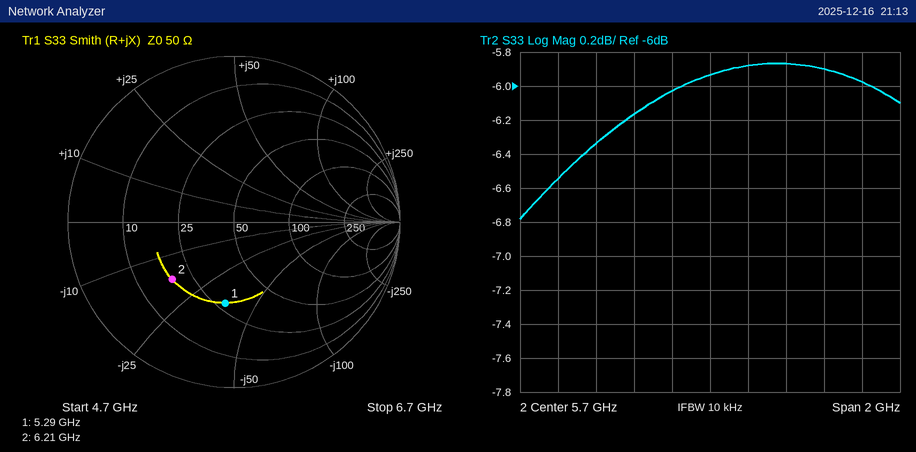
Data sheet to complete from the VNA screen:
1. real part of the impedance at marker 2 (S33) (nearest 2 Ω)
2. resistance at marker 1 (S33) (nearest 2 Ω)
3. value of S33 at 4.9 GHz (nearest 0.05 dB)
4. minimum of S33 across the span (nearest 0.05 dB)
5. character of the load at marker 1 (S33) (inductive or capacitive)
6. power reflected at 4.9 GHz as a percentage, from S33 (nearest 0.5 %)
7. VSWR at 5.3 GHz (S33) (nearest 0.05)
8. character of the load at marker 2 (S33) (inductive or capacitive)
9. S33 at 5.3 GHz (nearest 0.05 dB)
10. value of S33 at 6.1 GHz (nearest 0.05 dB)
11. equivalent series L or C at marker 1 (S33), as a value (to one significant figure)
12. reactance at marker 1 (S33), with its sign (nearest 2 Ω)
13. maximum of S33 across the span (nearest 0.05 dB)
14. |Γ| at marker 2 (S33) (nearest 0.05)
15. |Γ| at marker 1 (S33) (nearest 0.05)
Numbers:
18 Ω
28 Ω
-6.55 dB
-6.80 dB
capacitive
22.0 %
2.95
capacitive
-6.15 dB
-5.85 dB
800 fF
-36 Ω
-5.85 dB
0.50
0.50
